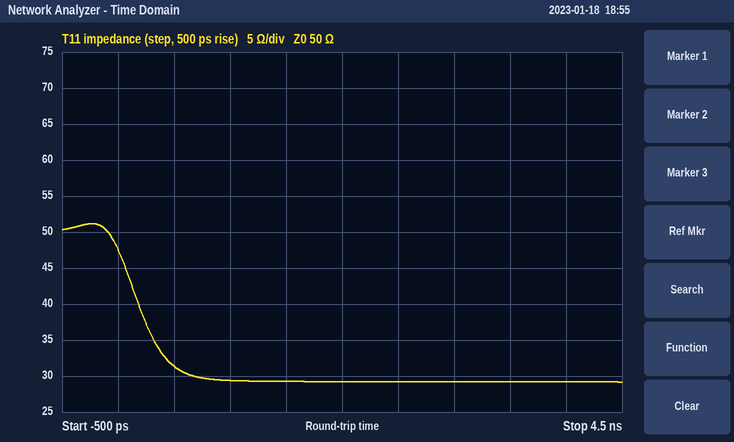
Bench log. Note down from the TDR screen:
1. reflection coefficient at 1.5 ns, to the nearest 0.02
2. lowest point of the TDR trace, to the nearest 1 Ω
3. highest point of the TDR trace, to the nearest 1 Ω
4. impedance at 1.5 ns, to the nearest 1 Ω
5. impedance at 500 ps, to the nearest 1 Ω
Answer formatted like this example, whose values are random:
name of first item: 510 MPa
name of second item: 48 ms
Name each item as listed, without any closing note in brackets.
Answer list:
reflection coefficient at 1.5 ns, to the nearest 0.02: -0.26
lowest point of the TDR trace, to the nearest 1 Ω: 29 Ω
highest point of the TDR trace, to the nearest 1 Ω: 51 Ω
impedance at 1.5 ns, to the nearest 1 Ω: 29 Ω
impedance at 500 ps, to the nearest 1 Ω: 31 Ω
